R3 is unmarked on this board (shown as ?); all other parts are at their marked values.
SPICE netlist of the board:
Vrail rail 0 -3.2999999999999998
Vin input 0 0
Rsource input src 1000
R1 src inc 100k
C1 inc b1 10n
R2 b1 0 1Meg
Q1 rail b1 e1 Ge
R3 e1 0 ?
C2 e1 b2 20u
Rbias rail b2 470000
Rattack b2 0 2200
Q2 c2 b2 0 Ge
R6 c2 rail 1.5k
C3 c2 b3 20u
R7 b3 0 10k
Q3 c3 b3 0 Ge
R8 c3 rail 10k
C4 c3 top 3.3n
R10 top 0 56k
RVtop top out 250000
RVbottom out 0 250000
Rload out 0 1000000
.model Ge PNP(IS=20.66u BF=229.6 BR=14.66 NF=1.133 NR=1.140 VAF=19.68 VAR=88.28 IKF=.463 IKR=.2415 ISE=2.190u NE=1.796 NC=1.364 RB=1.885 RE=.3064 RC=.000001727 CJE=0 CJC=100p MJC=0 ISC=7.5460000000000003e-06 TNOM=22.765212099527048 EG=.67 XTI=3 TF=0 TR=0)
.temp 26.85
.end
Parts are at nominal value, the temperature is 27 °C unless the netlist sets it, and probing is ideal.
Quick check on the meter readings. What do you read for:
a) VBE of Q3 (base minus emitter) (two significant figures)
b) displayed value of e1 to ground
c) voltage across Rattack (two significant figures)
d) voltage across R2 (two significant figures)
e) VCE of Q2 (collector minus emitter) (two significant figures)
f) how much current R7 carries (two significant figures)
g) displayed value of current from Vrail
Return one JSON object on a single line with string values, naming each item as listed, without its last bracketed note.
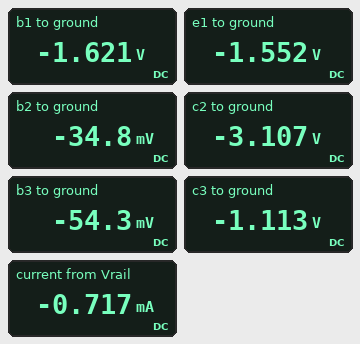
{"VBE of Q3 (base minus emitter)": "-54 mV", "displayed value of e1 to ground": "-1.552 V", "voltage across Rattack": "35 mV", "voltage across R2": "1.6 V", "VCE of Q2 (collector minus emitter)": "-3.1 V", "how much current R7 carries": "5.4 µA", "displayed value of current from Vrail": "-0.717 mA"}
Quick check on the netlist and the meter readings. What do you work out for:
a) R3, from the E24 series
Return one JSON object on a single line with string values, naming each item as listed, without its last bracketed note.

{"R3, from the E24 series": "4.3 kΩ"}
